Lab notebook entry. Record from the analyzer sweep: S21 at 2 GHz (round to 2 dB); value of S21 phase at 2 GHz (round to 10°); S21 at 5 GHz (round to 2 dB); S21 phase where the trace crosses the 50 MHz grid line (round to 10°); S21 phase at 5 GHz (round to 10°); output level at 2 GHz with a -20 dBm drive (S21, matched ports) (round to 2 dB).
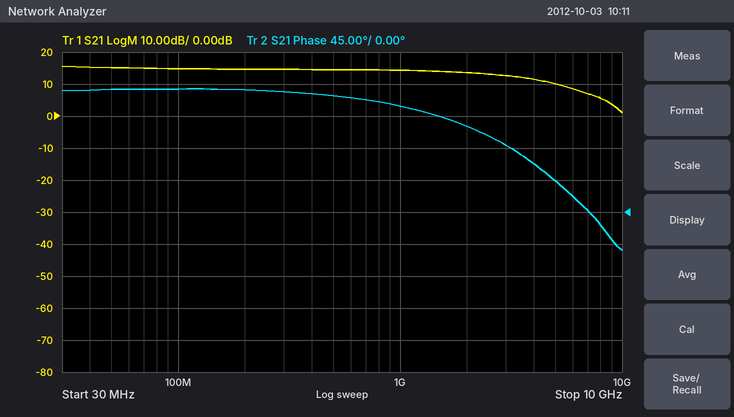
14 dB
120°
10 dB
170°
40°
-6 dBm
